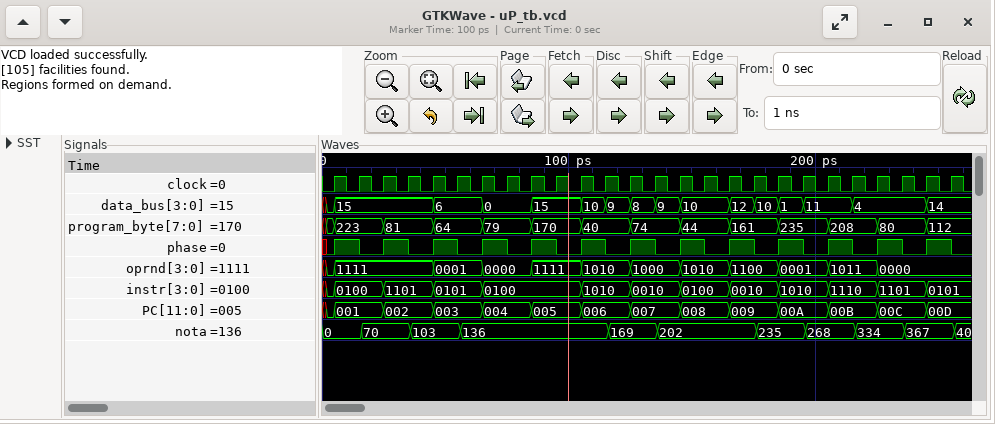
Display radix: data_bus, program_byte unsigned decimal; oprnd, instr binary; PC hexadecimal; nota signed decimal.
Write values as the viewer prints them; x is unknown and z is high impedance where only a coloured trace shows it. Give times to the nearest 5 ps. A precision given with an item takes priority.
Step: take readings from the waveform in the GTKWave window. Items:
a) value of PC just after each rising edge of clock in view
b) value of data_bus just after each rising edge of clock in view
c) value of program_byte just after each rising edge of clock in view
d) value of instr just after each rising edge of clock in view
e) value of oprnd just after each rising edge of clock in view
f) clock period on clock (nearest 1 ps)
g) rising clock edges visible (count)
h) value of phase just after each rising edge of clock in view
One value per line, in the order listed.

001, 001, 002, 002, 003, 003, 004, 004, 005, 005, 006, 006, 007, 007, 008, 008, 009, 009, 00A, 00A, 00B, 00B, 00C, 00C, 00D, 00D
15, 15, 15, 15, 6, 6, 0, 0, 15, 15, 10, 9, 8, 9, 10, 10, 12, 10, 1, 11, 11, 4, 4, 4, 14, 14
223, 223, 81, 81, 64, 64, 79, 79, 170, 170, 40, 40, 74, 74, 44, 44, 161, 161, 235, 235, 208, 208, 80, 80, 112, 112
0100, 0100, 1101, 1101, 0101, 0101, 0100, 0100, 0100, 0100, 1010, 1010, 0010, 0010, 0100, 0100, 0010, 0010, 1010, 1010, 1110, 1110, 1101, 1101, 0101, 0101
1111, 1111, 1111, 1111, 0001, 0001, 0000, 0000, 1111, 1111, 1010, 1010, 1000, 1000, 1010, 1010, 1100, 1100, 0001, 0001, 1011, 1011, 0000, 0000, 0000, 0000
10 ps
26
1 0 1 0 1 0 1 0 1 0 1 0 1 0 1 0 1 0 1 0 1 0 1 0 1 0
